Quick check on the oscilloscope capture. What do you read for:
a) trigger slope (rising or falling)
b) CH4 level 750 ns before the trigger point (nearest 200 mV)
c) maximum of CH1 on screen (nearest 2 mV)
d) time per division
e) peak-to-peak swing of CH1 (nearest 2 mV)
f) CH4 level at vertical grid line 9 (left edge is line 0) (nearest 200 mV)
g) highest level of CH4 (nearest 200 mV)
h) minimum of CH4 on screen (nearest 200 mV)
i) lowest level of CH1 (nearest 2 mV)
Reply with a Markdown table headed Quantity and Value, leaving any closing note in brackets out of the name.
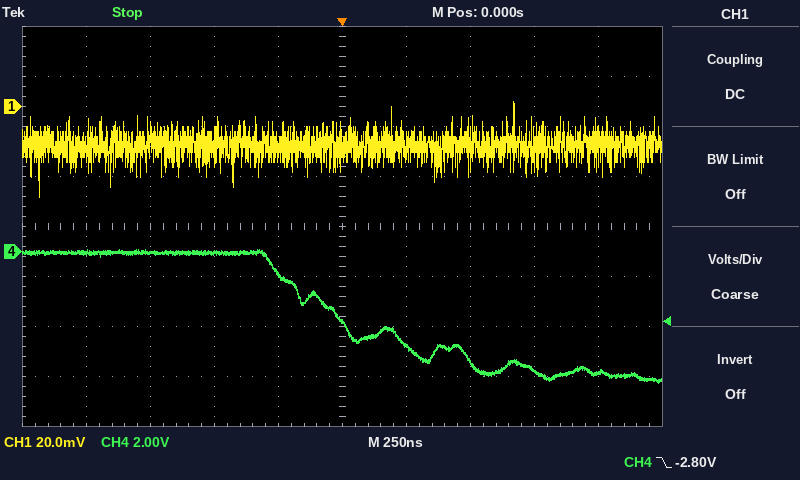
| Quantity | Value |
|---|---|
| trigger slope | falling |
| CH4 level 750 ns before the trigger point | 0.0 V |
| maximum of CH1 on screen | 2 mV |
| time per division | 250 ns |
| peak-to-peak swing of CH1 | 38 mV |
| CH4 level at vertical grid line 9 (left edge is line 0) | -4.8 V |
| highest level of CH4 | 0.0 V |
| minimum of CH4 on screen | -5.2 V |
| lowest level of CH1 | -36 mV |
